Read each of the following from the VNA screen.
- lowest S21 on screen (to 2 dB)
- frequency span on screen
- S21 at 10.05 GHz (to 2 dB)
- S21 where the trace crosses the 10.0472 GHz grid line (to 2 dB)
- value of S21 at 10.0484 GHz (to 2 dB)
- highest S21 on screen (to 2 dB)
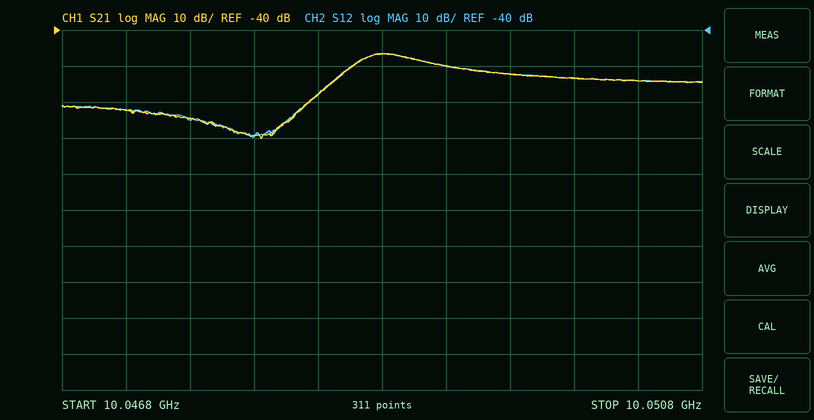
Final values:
-70 dB
4 MHz
-54 dB
-62 dB
-58 dB
-46 dB
